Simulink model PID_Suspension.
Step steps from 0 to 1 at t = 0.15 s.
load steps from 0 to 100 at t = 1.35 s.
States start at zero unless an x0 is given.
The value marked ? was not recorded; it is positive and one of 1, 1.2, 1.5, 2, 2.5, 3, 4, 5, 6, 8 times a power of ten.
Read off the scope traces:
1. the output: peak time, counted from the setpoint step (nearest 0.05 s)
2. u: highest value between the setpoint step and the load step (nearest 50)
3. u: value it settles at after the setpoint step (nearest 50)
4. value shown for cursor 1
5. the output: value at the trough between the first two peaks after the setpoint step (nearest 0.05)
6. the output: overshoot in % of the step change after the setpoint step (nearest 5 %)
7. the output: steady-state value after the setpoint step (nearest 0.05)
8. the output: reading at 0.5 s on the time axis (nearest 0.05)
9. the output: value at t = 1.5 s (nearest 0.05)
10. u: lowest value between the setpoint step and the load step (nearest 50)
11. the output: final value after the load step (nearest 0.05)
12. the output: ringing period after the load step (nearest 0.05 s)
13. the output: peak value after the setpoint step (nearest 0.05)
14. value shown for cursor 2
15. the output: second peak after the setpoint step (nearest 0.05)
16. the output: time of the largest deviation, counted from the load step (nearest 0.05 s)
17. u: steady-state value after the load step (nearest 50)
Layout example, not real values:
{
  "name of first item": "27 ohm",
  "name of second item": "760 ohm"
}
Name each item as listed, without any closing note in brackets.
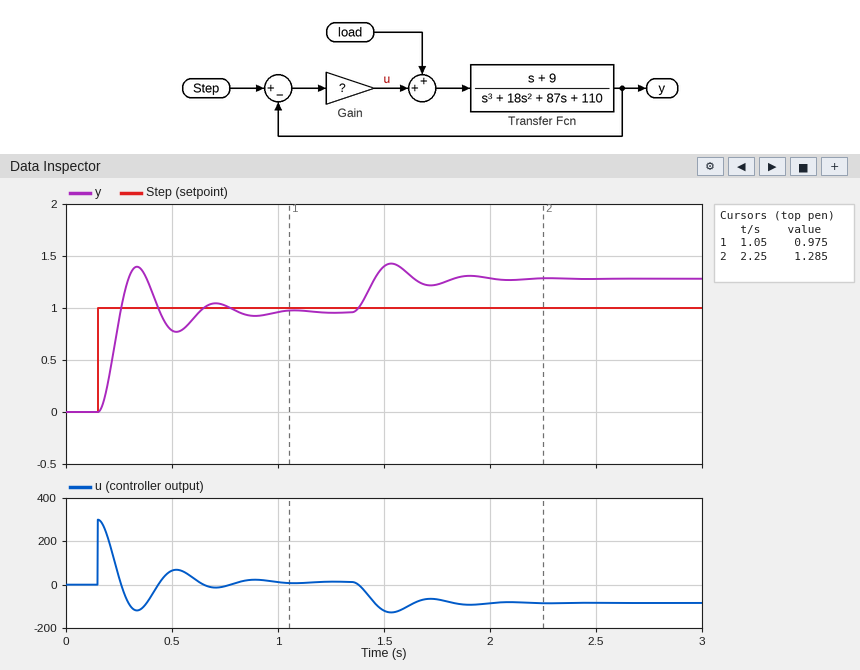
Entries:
{
  "the output: peak time, counted from the setpoint step": "0.20 s",
  "u: highest value between the setpoint step and the load step": "300",
  "u: value it settles at after the setpoint step": "0",
  "value shown for cursor 1": "0.975",
  "the output: value at the trough between the first two peaks after the setpoint step": "0.75",
  "the output: overshoot in % of the step change after the setpoint step": "45 %",
  "the output: steady-state value after the setpoint step": "0.95",
  "the output: reading at 0.5 s on the time axis": "0.80",
  "the output: value at t = 1.5 s": "1.40",
  "u: lowest value between the setpoint step and the load step": "-100",
  "the output: final value after the load step": "1.30",
  "the output: ringing period after the load step": "0.35 s",
  "the output: peak value after the setpoint step": "1.40",
  "value shown for cursor 2": "1.285",
  "the output: second peak after the setpoint step": "1.05",
  "the output: time of the largest deviation, counted from the load step": "0.20 s",
  "u: steady-state value after the load step": "-100"
}
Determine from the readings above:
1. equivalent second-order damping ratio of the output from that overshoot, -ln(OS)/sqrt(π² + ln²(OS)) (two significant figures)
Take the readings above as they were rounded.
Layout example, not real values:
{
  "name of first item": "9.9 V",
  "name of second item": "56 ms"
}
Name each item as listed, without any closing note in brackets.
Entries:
{
  "equivalent second-order damping ratio of the output from that overshoot, -ln(OS)/sqrt(π² + ln²(OS))": "0.25"
}
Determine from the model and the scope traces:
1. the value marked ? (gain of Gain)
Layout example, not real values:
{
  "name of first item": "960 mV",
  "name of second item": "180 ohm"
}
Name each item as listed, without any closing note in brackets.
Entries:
{
  "the value marked ?": "300"
}
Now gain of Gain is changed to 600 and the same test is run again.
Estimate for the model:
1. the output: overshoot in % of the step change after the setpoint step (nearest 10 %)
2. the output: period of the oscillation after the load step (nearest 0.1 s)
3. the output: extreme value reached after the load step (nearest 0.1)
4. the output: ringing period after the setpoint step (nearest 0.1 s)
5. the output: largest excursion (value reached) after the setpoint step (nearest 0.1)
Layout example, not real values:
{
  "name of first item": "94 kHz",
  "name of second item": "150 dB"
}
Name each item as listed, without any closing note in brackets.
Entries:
{
  "the output: overshoot in % of the step change after the setpoint step": "60 %",
  "the output: period of the oscillation after the load step": "0.3 s",
  "the output: extreme value reached after the load step": "1.2",
  "the output: ringing period after the setpoint step": "0.3 s",
  "the output: largest excursion (value reached) after the setpoint step": "1.5"
}
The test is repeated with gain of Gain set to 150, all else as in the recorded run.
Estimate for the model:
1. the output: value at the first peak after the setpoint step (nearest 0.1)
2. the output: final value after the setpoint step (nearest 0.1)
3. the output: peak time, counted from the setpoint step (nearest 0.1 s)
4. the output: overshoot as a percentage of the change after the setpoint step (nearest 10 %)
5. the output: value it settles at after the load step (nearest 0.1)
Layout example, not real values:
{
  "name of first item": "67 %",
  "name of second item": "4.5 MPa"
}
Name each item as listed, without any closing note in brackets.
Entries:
{
  "the output: value at the first peak after the setpoint step": "1.2",
  "the output: final value after the setpoint step": "0.9",
  "the output: peak time, counted from the setpoint step": "0.3 s",
  "the output: overshoot as a percentage of the change after the setpoint step": "30 %",
  "the output: value it settles at after the load step": "1.5"
}
